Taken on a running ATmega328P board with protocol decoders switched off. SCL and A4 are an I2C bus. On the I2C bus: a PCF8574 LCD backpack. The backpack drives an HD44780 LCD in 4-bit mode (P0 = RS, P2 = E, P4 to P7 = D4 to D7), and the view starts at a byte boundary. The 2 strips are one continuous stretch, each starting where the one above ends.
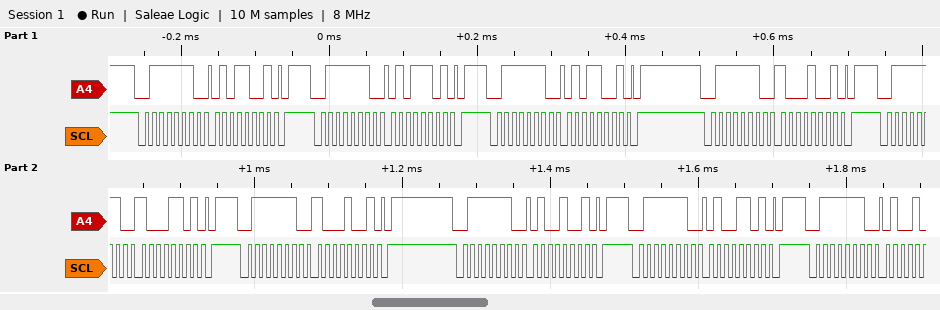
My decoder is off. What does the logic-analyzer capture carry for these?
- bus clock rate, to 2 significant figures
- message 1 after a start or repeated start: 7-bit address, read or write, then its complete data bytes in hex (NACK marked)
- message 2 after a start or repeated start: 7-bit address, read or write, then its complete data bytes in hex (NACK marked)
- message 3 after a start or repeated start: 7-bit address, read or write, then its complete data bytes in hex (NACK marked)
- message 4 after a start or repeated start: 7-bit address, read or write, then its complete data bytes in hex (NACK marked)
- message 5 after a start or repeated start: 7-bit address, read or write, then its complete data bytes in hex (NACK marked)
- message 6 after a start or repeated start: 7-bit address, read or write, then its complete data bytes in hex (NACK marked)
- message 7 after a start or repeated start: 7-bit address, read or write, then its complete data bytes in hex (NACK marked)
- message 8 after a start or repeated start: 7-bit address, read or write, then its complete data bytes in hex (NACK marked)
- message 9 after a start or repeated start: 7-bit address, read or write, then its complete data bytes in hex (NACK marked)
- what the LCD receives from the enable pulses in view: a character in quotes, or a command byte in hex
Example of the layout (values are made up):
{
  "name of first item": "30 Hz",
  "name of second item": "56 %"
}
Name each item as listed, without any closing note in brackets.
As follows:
{
  "bus clock rate, to 2 significant figures": "100 kHz",
  "message 1 after a start or repeated start: 7-bit address, read or write, then its complete data bytes in hex": "0x3F write: 59",
  "message 2 after a start or repeated start: 7-bit address, read or write, then its complete data bytes in hex": "0x3F write: 5D",
  "message 3 after a start or repeated start: 7-bit address, read or write, then its complete data bytes in hex": "0x3F write: 59",
  "message 4 after a start or repeated start: 7-bit address, read or write, then its complete data bytes in hex": "0x3F write: 89",
  "message 5 after a start or repeated start: 7-bit address, read or write, then its complete data bytes in hex": "0x3F write: 8D",
  "message 6 after a start or repeated start: 7-bit address, read or write, then its complete data bytes in hex": "0x3F write: 89",
  "message 7 after a start or repeated start: 7-bit address, read or write, then its complete data bytes in hex": "0x3F write: 49",
  "message 8 after a start or repeated start: 7-bit address, read or write, then its complete data bytes in hex": "0x3F write: 4D",
  "message 9 after a start or repeated start: 7-bit address, read or write, then its complete data bytes in hex": "0x3F write",
  "what the LCD receives from the enable pulses in view: a character in quotes, or a command byte in hex": "'X'"
}
